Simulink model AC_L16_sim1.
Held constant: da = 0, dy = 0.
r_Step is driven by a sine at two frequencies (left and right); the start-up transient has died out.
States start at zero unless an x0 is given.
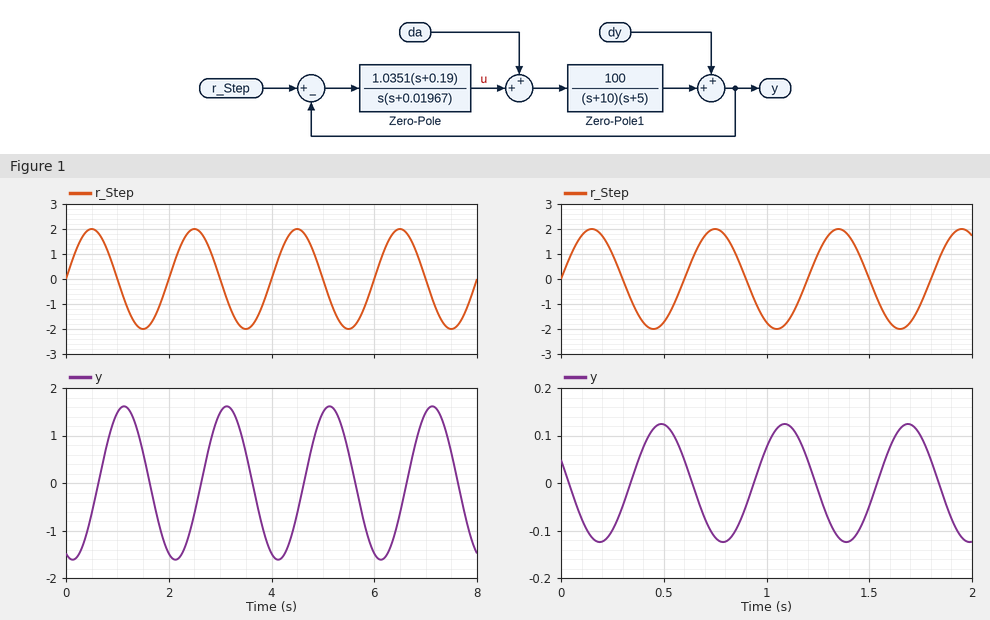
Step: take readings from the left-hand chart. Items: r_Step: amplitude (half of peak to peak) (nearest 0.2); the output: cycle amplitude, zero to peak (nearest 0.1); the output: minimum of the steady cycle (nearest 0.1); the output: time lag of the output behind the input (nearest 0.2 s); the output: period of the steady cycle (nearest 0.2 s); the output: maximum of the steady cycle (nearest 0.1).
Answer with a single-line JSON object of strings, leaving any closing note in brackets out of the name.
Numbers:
{"r_Step: amplitude (half of peak to peak)": "2.0", "the output: cycle amplitude, zero to peak": "1.6", "the output: minimum of the steady cycle": "-1.6", "the output: time lag of the output behind the input": "0.6 s", "the output: period of the steady cycle": "2.0 s", "the output: maximum of the steady cycle": "1.6"}
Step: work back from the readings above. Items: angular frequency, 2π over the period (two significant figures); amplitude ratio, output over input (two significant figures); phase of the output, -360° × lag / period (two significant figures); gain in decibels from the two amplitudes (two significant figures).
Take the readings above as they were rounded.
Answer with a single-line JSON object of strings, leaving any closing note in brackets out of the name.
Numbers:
{"angular frequency, 2π over the period": "3.1 rad/s", "amplitude ratio, output over input": "0.80", "phase of the output, -360° × lag / period": "-110°", "gain in decibels from the two amplitudes": "-1.9 dB"}
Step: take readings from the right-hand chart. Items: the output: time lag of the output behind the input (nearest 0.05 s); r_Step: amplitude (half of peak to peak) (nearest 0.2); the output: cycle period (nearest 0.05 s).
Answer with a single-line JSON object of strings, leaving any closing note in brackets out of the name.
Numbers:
{"the output: time lag of the output behind the input": "0.35 s", "r_Step: amplitude (half of peak to peak)": "2.0", "the output: cycle period": "0.60 s"}
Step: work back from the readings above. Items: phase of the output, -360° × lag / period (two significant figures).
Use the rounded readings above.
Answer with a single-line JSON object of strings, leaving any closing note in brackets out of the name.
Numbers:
{"phase of the output, -360° × lag / period": "-210°"}
